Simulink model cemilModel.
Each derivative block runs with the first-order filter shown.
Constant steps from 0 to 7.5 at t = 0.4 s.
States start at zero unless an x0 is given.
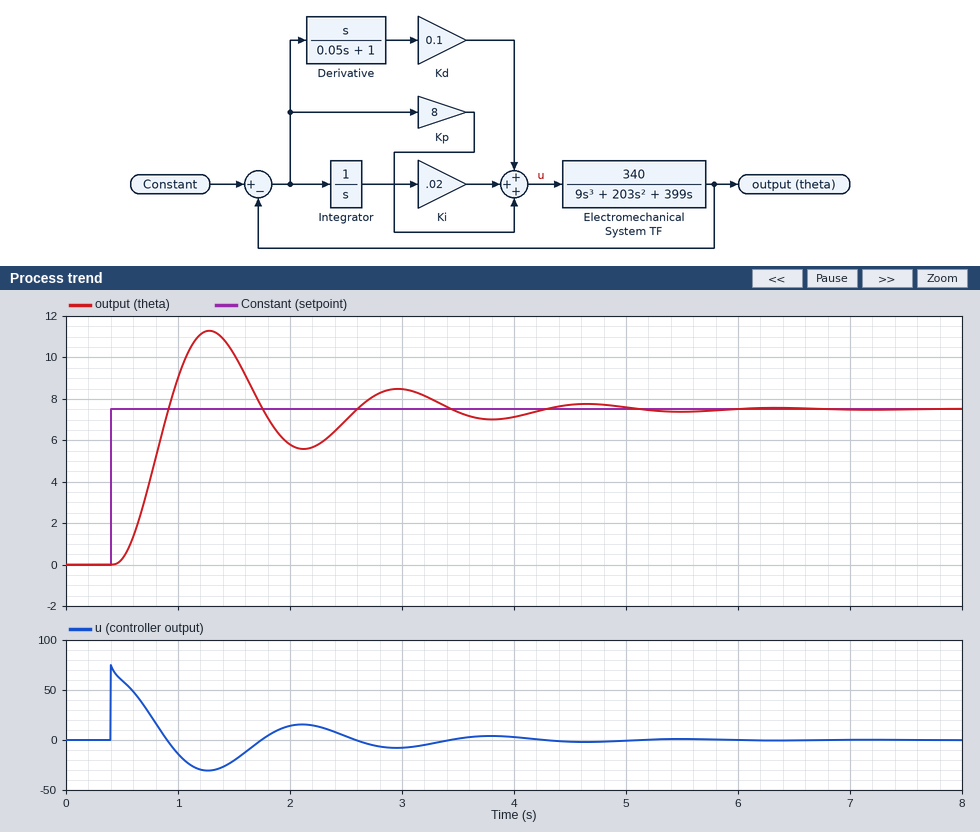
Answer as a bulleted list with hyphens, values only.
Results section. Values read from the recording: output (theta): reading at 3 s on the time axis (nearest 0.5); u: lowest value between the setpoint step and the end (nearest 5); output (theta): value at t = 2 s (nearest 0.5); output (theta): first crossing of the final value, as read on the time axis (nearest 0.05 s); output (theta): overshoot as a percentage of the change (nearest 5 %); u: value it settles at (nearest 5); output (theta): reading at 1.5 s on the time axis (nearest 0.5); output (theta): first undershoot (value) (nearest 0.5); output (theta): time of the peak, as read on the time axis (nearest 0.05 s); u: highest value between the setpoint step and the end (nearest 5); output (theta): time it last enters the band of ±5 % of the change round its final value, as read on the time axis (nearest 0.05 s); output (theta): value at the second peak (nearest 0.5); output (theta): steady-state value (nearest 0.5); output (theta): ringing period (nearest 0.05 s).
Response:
- 8.5
- -30
- 6.0
- 0.90 s
- 50 %
- 0
- 10.0
- 5.5
- 1.30 s
- 75
- 4.00 s
- 8.5
- 7.5
- 1.70 s
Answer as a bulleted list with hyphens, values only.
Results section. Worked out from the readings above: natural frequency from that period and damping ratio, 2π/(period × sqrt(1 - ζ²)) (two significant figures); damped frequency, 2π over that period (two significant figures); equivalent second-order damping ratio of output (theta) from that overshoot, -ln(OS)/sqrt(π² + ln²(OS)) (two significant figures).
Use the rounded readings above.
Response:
- 3.8 rad/s
- 3.7 rad/s
- 0.22
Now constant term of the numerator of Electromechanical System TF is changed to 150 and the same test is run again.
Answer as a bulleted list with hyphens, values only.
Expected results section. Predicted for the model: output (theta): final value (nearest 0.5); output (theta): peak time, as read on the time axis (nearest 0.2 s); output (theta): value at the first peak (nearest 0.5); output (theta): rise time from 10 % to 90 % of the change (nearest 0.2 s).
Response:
- 7.5
- 1.8 s
- 9.5
- 0.6 s
